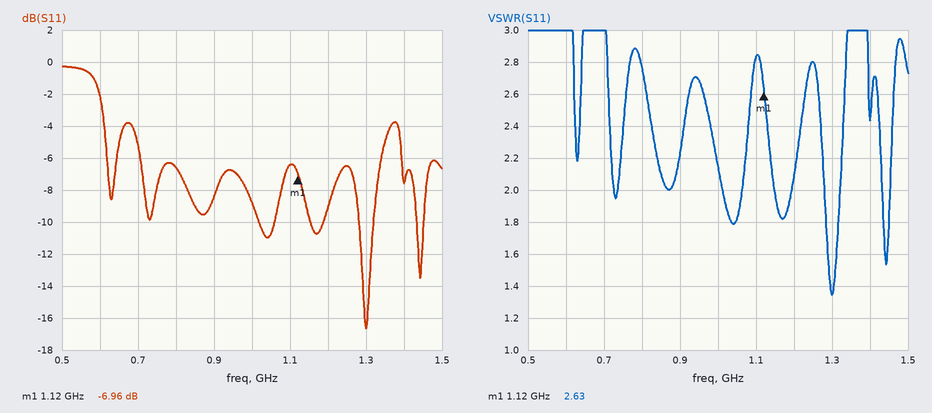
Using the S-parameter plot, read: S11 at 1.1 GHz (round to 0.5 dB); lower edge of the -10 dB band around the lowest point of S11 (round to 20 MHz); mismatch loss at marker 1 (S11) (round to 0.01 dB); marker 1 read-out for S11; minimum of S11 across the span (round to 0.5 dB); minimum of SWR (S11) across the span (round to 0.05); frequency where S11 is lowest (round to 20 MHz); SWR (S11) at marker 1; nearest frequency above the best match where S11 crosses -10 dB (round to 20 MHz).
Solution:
-6.5 dB
1.28 GHz
0.98 dB
-6.96 dB
-16.5 dB
1.35
1.30 GHz
2.63
1.32 GHz
